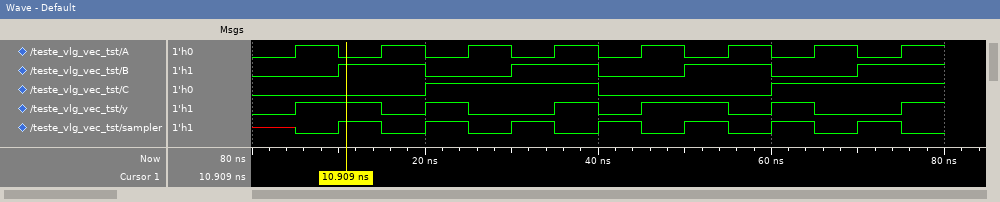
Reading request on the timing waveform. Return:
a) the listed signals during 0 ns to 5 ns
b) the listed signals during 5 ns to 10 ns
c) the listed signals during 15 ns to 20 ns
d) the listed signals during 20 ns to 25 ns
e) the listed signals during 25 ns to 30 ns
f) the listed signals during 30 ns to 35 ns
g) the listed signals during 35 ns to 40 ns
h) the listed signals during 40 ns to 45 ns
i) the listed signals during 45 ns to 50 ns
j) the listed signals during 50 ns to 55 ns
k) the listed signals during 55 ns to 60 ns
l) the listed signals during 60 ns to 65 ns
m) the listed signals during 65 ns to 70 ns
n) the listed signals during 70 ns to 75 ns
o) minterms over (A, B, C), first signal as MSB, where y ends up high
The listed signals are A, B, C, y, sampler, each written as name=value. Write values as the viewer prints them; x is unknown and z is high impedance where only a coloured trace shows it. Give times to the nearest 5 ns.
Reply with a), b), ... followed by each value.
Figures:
a) A=0, B=0, C=0, y=0, sampler=x
b) A=1, B=0, C=0, y=1, sampler=0
c) A=1, B=1, C=0, y=0, sampler=0
d) A=0, B=0, C=1, y=1, sampler=1
e) A=1, B=0, C=1, y=0, sampler=0
f) A=0, B=1, C=1, y=0, sampler=1
g) A=1, B=1, C=1, y=1, sampler=0
h) A=0, B=0, C=0, y=0, sampler=1
i) A=1, B=0, C=0, y=1, sampler=0
j) A=0, B=1, C=0, y=1, sampler=1
k) A=1, B=1, C=0, y=0, sampler=0
l) A=0, B=0, C=1, y=1, sampler=1
m) A=1, B=0, C=1, y=0, sampler=0
n) A=0, B=1, C=1, y=0, sampler=1
o) 1, 2, 4, 7
